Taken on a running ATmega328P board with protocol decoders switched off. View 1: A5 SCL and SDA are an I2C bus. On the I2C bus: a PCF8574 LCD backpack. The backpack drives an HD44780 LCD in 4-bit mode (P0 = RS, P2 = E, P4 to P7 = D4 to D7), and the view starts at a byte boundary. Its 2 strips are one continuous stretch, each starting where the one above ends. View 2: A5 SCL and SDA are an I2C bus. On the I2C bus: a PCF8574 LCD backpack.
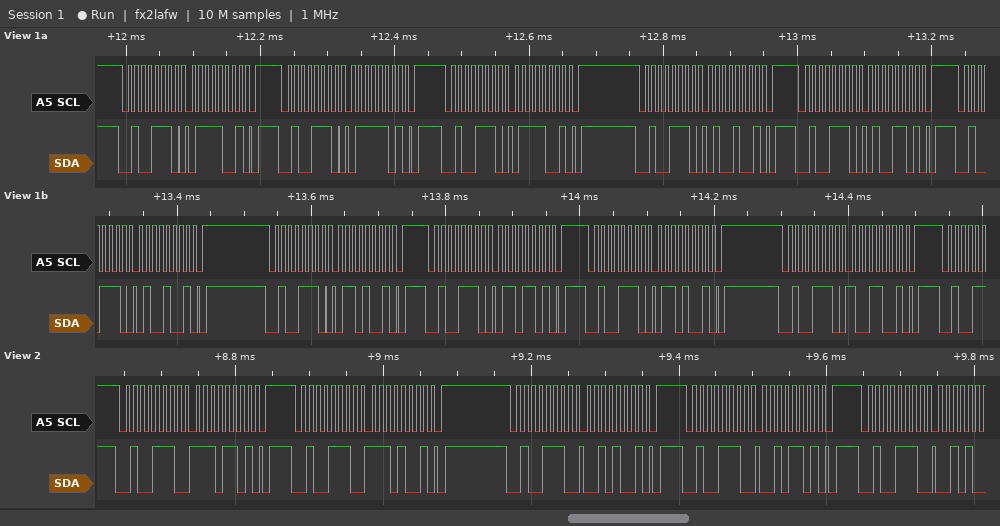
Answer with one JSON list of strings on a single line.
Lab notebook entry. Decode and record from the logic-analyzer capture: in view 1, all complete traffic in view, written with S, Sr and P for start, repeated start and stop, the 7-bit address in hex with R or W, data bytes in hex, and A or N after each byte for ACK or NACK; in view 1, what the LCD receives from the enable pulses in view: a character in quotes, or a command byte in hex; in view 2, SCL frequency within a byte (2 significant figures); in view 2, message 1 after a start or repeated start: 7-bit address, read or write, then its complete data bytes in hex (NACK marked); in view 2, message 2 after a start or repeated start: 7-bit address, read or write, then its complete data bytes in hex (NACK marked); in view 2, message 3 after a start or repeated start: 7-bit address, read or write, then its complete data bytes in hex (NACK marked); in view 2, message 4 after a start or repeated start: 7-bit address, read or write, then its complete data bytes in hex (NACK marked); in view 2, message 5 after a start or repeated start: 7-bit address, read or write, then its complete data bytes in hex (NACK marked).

["S 27W A 79 A P S 27W A 7D A P S 27W A 79 A P S 27W A 49 A P S 27W A 4D A P S 27W A 49 A P S 27W A 69 A P S 27W A 6D A P S 27W A 69 A P S 27W A 99 A P", "'t'", "100 kHz", "0x27 write: ED", "0x27 write: E9", "0x27 write: 29", "0x27 write: 2D", "0x27 write"]
